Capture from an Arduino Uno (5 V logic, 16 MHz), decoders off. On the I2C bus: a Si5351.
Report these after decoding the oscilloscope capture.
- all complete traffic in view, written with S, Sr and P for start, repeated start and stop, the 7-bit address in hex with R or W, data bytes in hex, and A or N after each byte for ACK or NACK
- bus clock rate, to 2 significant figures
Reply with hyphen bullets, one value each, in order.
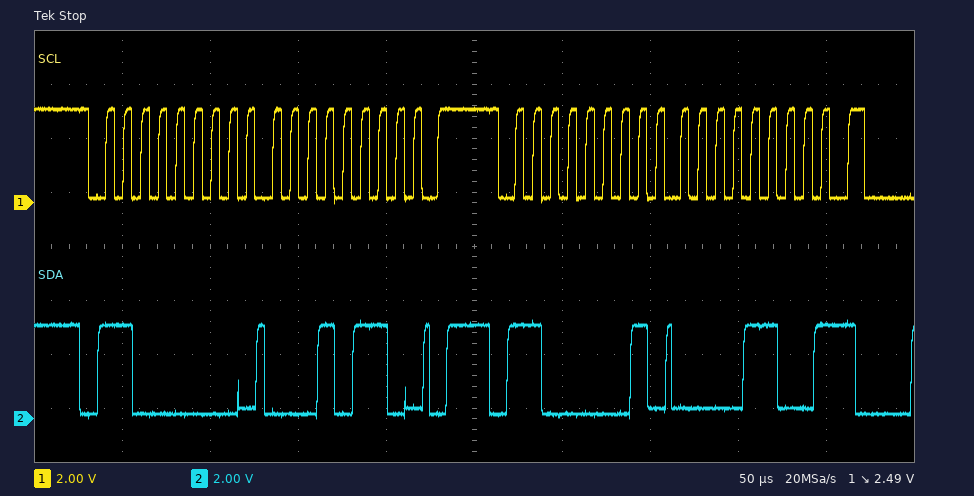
- S 60W A 16 A P S 60R A 0C N
- 100 kHz
